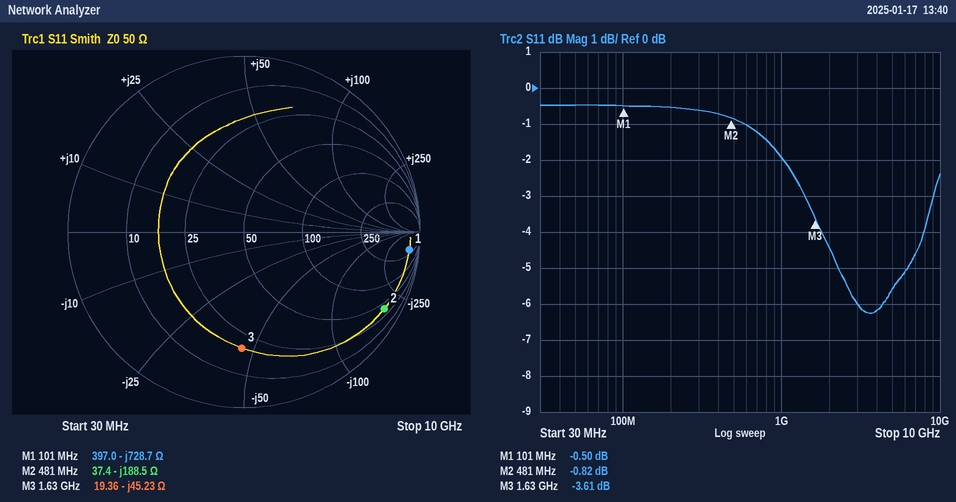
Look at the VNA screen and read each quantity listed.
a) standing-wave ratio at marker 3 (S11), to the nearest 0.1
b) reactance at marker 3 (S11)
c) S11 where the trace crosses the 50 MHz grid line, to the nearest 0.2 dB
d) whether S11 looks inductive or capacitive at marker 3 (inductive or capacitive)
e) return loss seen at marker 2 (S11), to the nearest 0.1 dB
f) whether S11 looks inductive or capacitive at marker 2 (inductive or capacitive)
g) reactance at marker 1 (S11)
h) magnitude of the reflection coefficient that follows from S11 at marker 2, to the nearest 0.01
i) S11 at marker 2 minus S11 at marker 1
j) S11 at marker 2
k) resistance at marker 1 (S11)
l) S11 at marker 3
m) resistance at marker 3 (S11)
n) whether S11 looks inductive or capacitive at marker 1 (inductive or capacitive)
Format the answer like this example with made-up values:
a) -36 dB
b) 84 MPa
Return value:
a) 4.9
b) -45.23 Ω
c) -0.4 dB
d) capacitive
e) 0.8 dB
f) capacitive
g) -728.7 Ω
h) 0.91
i) -0.32 dB
j) -0.82 dB
k) 397.0 Ω
l) -3.61 dB
m) 19.36 Ω
n) capacitive
